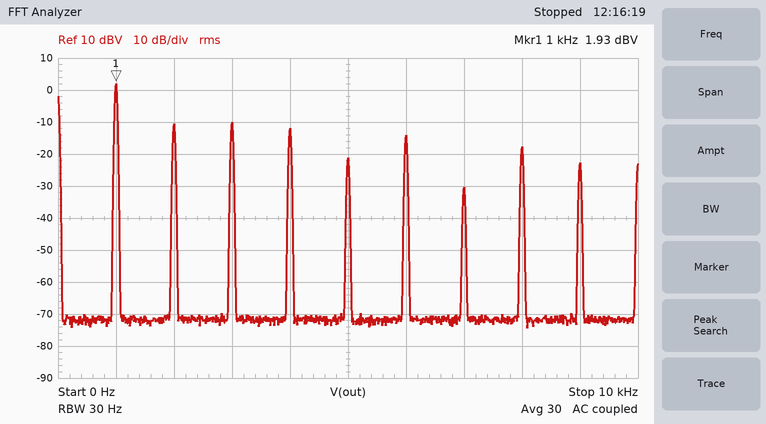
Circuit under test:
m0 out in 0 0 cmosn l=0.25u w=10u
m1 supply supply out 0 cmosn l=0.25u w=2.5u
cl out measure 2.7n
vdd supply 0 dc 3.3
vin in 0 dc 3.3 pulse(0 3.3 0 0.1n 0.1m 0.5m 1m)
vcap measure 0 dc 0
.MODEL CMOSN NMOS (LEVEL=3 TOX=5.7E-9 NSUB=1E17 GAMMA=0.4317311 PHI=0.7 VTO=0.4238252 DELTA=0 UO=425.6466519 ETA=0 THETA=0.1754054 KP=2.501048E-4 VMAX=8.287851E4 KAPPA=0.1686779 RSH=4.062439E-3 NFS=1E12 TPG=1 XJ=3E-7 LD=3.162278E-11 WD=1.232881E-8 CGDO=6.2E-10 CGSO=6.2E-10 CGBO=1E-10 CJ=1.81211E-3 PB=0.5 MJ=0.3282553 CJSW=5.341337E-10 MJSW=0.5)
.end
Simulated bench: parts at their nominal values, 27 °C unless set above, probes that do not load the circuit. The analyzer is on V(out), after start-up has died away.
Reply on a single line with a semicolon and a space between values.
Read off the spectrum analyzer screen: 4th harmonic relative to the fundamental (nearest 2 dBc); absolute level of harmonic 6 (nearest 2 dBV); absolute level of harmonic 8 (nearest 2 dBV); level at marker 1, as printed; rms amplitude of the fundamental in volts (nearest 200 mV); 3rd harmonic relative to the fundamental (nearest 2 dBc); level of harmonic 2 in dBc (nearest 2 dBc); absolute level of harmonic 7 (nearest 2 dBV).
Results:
-14 dBc; -14 dBV; -18 dBV; 1.93 dBV; 1.2 V; -12 dBc; -12 dBc; -30 dBV
